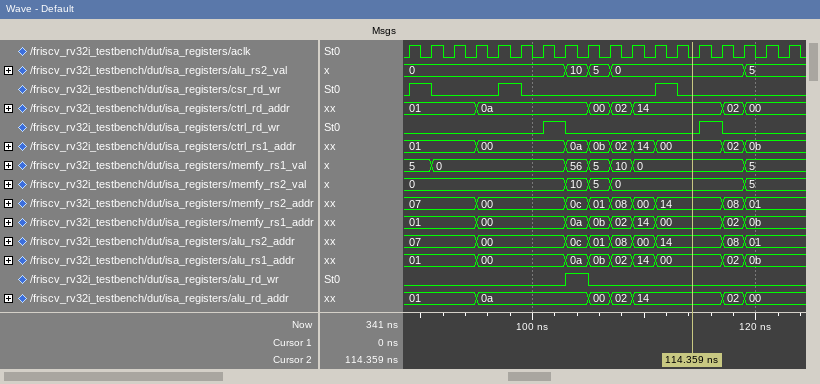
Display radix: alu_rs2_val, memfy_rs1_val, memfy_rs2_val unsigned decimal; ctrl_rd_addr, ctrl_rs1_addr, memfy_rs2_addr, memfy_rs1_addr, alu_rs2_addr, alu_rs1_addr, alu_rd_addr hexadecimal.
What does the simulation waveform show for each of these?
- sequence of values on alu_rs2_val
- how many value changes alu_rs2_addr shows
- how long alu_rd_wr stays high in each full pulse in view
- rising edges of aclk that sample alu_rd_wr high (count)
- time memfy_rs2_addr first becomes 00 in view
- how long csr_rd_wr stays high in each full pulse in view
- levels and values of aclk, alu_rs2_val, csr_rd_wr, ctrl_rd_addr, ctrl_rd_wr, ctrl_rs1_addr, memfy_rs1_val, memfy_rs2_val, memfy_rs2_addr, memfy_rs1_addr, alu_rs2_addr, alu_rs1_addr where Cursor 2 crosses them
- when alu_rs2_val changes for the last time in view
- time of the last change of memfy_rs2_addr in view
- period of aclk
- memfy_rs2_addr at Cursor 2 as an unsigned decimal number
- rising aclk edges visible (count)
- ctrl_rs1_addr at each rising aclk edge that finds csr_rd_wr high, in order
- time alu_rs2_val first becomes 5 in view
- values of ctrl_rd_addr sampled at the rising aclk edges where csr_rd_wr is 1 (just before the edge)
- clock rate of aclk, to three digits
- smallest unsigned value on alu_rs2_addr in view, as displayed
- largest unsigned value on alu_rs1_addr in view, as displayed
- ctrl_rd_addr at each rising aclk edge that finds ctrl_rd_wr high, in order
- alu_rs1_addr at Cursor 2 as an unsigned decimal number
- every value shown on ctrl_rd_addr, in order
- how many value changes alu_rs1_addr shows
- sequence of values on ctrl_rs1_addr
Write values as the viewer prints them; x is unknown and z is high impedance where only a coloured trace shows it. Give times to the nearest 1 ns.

0, 10, 5, 0, 5
8
2 ns
1
95 ns
2 ns, 2 ns, 2 ns
aclk=0, alu_rs2_val=0, csr_rd_wr=0, ctrl_rd_addr=14, ctrl_rd_wr=0, ctrl_rs1_addr=00, memfy_rs1_val=0, memfy_rs2_val=0, memfy_rs2_addr=14, memfy_rs1_addr=00, alu_rs2_addr=14, alu_rs1_addr=00
119 ns
119 ns
2 ns
20
18
01, 00, 00
105 ns
01, 0a, 14
500 MHz
00
14
0a, 14
0
01, 0a, 00, 02, 14, 02, 00
8
01, 00, 0a, 0b, 02, 14, 00, 02, 0b
